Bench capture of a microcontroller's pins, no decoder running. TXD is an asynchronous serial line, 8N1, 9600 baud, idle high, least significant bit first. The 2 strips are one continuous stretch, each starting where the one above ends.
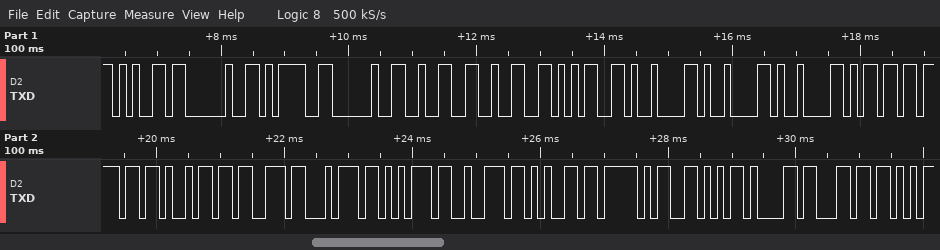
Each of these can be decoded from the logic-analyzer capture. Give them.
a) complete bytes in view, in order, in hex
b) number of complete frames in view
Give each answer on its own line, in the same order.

0x65 0x20 0x3D 0x20 0x32 0x32 0x35 0x09 0x09 0x09 0x6D 0x6F 0x69 0x73 0x74 0x75 0x72 0x65 0x5F 0x56 0x61 0x6C
22
